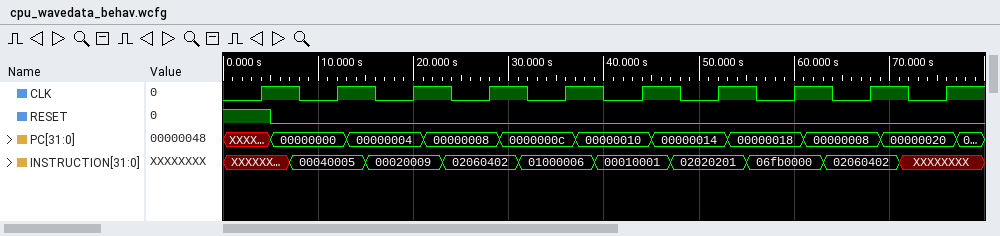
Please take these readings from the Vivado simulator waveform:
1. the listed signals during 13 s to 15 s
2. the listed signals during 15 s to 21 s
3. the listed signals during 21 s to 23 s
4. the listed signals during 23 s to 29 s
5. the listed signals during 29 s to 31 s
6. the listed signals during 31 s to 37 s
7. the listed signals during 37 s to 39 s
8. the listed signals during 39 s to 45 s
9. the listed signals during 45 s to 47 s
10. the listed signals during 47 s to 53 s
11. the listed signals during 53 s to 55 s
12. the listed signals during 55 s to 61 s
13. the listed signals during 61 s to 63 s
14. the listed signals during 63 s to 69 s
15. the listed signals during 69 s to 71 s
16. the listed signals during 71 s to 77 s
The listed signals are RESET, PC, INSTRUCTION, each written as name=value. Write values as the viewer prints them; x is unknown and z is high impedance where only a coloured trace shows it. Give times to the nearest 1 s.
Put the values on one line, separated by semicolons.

RESET=0, PC=00000004, INSTRUCTION=00040005; RESET=0, PC=00000004, INSTRUCTION=00020009; RESET=0, PC=00000008, INSTRUCTION=00020009; RESET=0, PC=00000008, INSTRUCTION=02060402; RESET=0, PC=0000000c, INSTRUCTION=02060402; RESET=0, PC=0000000c, INSTRUCTION=01000006; RESET=0, PC=00000010, INSTRUCTION=01000006; RESET=0, PC=00000010, INSTRUCTION=00010001; RESET=0, PC=00000014, INSTRUCTION=00010001; RESET=0, PC=00000014, INSTRUCTION=02020201; RESET=0, PC=00000018, INSTRUCTION=02020201; RESET=0, PC=00000018, INSTRUCTION=06fb0000; RESET=0, PC=00000008, INSTRUCTION=06fb0000; RESET=0, PC=00000008, INSTRUCTION=02060402; RESET=0, PC=00000020, INSTRUCTION=02060402; RESET=0, PC=00000020, INSTRUCTION=XXXXXXXX
